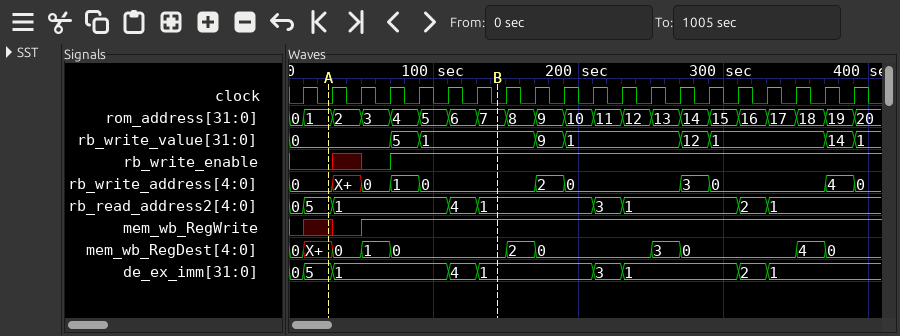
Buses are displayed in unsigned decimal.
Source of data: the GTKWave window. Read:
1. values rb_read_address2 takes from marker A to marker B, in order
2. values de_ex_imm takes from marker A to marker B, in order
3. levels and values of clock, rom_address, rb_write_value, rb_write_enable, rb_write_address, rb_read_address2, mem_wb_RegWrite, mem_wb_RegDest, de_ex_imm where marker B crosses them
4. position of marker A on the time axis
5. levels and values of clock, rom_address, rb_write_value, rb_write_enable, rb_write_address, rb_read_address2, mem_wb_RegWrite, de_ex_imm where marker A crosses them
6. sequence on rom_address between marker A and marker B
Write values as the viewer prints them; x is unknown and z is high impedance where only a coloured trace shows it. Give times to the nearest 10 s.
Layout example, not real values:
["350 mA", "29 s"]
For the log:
["5, 1, 4, 1", "5, 1, 4, 1", "clock=0, rom_address=7, rb_write_value=1, rb_write_enable=1, rb_write_address=0, rb_read_address2=1, mem_wb_RegWrite=1, mem_wb_RegDest=0, de_ex_imm=1", "30 s", "clock=0, rom_address=1, rb_write_value=0, rb_write_enable=0, rb_write_address=0, rb_read_address2=5, mem_wb_RegWrite=x, de_ex_imm=5", "1, 2, 3, 4, 5, 6, 7"]
